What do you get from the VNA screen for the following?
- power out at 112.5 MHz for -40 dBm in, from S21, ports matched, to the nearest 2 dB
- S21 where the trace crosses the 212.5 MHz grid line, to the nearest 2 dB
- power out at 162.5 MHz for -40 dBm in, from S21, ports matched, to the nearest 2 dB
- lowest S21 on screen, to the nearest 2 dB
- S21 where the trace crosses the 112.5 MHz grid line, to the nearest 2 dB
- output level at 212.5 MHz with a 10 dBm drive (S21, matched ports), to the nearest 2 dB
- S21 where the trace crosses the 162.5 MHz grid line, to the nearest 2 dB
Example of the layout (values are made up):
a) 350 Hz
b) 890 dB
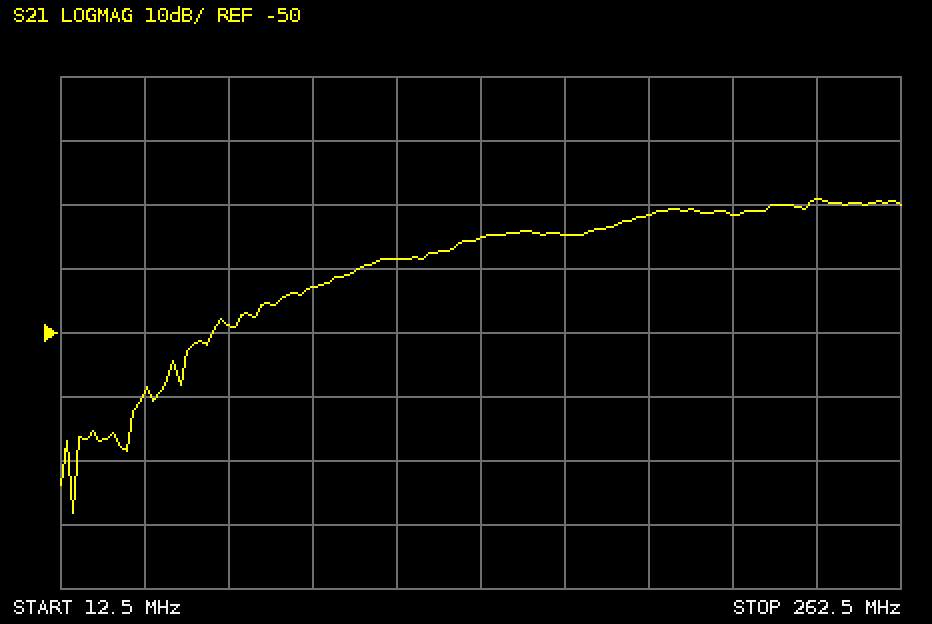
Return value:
a) -78 dBm
b) -32 dB
c) -74 dBm
d) -78 dB
e) -38 dB
f) -22 dBm
g) -34 dB
